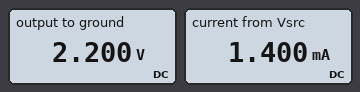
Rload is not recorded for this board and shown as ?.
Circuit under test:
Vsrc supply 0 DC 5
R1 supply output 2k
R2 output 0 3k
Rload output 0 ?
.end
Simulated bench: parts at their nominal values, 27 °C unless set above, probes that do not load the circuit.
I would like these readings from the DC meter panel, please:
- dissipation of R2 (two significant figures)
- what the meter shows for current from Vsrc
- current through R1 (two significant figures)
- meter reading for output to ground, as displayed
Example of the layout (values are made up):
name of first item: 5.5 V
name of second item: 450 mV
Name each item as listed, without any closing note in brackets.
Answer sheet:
dissipation of R2: 1.6 mW
what the meter shows for current from Vsrc: 1.400 mA
current through R1: 1.4 mA
meter reading for output to ground, as displayed: 2.200 V
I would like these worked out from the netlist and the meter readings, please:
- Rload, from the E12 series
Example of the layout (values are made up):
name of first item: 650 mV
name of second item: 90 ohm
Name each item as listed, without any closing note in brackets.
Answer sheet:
Rload, from the E12 series: 3.3 kΩ
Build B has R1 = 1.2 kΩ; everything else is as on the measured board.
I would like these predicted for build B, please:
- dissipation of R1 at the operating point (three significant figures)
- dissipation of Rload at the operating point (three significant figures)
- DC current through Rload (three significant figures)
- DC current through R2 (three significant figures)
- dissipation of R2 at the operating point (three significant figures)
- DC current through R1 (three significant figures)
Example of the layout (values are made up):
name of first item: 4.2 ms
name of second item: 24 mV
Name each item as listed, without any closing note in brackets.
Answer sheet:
dissipation of R1 at the operating point: 3.91 mW
dissipation of Rload at the operating point: 2.44 mW
DC current through Rload: 859 µA
DC current through R2: 945 µA
dissipation of R2 at the operating point: 2.68 mW
DC current through R1: 1.80 mA
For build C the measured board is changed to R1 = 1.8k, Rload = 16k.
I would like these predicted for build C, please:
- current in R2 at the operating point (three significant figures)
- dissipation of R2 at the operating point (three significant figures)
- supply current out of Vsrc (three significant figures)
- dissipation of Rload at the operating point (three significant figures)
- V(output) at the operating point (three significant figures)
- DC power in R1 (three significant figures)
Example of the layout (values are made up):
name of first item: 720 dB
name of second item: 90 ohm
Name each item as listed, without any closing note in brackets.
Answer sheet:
current in R2 at the operating point: 973 µA
dissipation of R2 at the operating point: 2.84 mW
supply current out of Vsrc: 1.16 mA
dissipation of Rload at the operating point: 533 µW
V(output) at the operating point: 2.92 V
DC power in R1: 2.40 mW
